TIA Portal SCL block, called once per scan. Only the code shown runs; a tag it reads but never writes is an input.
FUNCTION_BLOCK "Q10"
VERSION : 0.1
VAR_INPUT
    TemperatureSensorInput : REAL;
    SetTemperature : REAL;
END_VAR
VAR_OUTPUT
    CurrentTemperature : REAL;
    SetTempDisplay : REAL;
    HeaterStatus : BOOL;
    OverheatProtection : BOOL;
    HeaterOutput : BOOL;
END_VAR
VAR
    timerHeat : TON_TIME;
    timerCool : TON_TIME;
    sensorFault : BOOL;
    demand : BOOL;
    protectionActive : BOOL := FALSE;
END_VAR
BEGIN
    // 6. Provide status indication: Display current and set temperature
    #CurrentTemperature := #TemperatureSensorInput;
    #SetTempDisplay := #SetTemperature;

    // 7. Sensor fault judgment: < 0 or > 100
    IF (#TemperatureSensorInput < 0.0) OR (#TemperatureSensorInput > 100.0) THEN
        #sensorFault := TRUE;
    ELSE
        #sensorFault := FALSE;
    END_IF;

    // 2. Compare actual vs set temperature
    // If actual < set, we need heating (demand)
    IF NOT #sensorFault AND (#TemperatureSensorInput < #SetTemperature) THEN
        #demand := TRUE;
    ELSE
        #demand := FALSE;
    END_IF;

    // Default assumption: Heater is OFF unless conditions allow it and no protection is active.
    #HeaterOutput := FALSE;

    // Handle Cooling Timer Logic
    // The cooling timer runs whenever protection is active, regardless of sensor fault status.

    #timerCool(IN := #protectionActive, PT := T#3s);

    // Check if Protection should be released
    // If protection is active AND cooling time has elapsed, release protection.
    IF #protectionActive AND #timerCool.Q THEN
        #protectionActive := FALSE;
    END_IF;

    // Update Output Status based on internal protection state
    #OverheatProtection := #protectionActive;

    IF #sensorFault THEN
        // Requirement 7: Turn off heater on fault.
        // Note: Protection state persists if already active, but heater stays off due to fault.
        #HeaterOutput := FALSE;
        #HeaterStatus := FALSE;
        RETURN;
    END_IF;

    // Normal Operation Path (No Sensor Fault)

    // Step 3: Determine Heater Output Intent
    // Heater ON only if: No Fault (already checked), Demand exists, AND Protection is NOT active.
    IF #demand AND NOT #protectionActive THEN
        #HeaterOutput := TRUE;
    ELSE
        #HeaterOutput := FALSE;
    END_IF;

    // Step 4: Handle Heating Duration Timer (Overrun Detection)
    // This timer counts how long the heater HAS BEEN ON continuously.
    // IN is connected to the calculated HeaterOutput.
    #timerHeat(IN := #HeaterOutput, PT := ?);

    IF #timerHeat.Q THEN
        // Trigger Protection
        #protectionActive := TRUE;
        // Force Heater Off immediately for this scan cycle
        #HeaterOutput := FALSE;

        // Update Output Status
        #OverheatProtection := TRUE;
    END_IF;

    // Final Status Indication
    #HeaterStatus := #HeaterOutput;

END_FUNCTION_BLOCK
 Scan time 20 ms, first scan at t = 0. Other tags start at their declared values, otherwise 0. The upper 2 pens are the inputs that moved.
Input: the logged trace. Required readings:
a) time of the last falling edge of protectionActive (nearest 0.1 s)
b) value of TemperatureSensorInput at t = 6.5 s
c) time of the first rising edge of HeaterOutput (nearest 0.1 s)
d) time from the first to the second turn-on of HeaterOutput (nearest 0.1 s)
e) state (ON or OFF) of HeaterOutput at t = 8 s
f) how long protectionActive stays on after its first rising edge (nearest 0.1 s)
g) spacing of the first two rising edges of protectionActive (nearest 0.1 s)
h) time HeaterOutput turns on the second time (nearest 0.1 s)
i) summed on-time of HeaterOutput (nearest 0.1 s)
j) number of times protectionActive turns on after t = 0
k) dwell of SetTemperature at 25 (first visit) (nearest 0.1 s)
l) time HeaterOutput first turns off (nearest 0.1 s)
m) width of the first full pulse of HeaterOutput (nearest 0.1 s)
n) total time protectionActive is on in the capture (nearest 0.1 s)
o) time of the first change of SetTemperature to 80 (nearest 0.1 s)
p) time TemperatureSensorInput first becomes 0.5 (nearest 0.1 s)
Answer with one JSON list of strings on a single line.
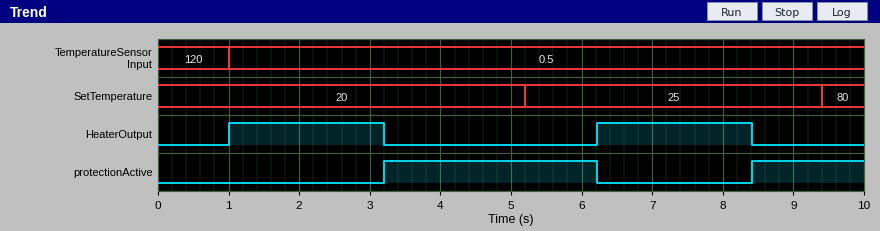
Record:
["6.2 s", "0.5", "1.0 s", "5.2 s", "ON", "3.0 s", "5.2 s", "6.2 s", "4.4 s", "2", "4.2 s", "3.2 s", "2.2 s", "4.6 s", "9.4 s", "1.0 s"]
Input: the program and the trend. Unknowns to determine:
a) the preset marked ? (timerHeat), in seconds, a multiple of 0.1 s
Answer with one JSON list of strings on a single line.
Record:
["2.2 s"]
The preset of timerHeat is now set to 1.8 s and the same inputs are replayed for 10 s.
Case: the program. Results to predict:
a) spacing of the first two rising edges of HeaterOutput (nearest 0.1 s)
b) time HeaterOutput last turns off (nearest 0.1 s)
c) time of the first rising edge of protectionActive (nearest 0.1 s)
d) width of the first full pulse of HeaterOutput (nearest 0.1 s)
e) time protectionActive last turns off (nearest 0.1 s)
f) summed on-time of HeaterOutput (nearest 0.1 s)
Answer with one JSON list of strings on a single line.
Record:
["4.8 s", "7.6 s", "2.8 s", "1.8 s", "5.8 s", "3.6 s"]
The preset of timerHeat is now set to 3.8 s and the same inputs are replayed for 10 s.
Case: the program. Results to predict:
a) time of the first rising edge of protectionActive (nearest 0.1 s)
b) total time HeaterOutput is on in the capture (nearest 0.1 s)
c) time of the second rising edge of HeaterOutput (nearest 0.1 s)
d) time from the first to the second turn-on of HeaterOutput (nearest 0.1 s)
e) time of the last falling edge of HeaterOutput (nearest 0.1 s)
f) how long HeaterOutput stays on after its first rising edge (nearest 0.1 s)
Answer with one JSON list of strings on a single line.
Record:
["4.8 s", "6.0 s", "7.8 s", "6.8 s", "4.8 s", "3.8 s"]
